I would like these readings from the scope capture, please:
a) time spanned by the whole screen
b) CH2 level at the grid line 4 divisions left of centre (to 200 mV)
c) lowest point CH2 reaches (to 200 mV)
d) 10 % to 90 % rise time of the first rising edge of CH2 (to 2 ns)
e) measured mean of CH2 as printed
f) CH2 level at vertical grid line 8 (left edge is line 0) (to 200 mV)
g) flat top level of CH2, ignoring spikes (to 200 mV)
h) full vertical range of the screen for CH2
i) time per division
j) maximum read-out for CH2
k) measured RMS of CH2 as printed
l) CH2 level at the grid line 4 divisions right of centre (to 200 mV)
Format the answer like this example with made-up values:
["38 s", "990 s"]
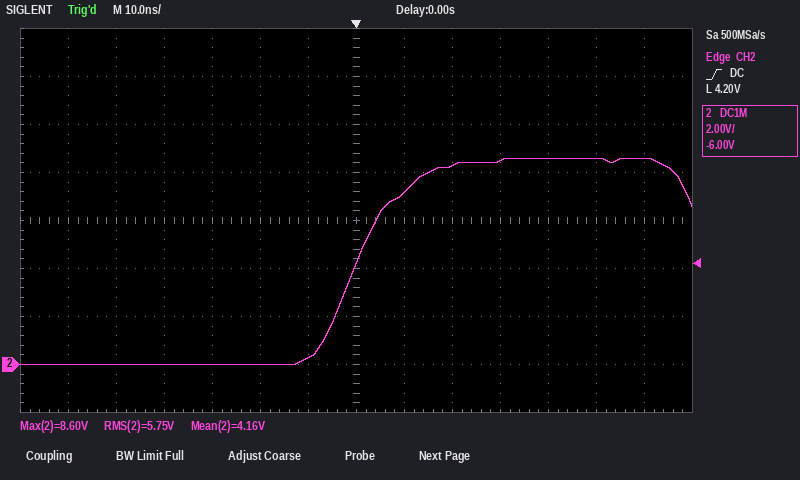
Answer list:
["140 ns", "0.0 V", "0.0 V", "20 ns", "4.16 V", "7.2 V", "8.6 V", "16 V", "10 ns", "8.60 V", "5.75 V", "8.6 V"]
